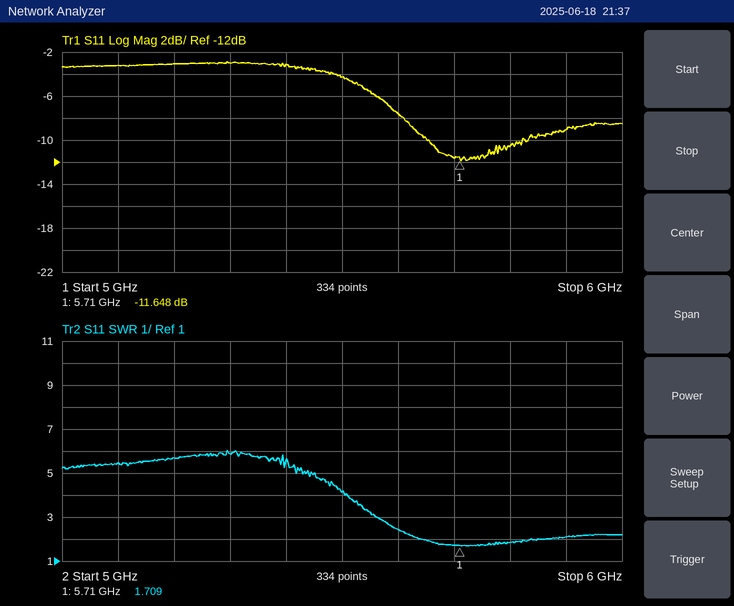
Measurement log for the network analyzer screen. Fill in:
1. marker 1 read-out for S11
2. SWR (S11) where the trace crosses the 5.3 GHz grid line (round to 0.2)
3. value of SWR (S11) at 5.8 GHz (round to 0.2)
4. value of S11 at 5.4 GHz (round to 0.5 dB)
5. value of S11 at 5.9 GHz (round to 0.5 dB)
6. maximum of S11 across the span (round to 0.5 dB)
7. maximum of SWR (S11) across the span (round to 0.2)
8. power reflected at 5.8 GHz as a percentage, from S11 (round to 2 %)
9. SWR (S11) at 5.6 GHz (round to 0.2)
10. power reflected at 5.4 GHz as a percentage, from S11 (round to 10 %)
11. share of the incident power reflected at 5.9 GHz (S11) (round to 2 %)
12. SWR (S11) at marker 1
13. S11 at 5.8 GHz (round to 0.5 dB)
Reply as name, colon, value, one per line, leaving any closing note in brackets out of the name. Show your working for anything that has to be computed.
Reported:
marker 1 read-out for S11: -11.648 dB
SWR (S11) where the trace crosses the 5.3 GHz grid line: 5.8
value of SWR (S11) at 5.8 GHz: 1.8
value of S11 at 5.4 GHz: -3.0 dB
value of S11 at 5.9 GHz: -9.0 dB
maximum of S11 across the span: -3.0 dB
maximum of SWR (S11) across the span: 6.0
power reflected at 5.8 GHz as a percentage, from S11: 10^(-10.5/10) ≈ 8.91 %, so 8 % to the nearest 2 %
SWR (S11) at 5.6 GHz: 2.4
power reflected at 5.4 GHz as a percentage, from S11: 10^(-3/10) ≈ 50 %
share of the incident power reflected at 5.9 GHz (S11): 10^(-9/10) ≈ 12.6 %, so 12 % to the nearest 2 %
SWR (S11) at marker 1: 1.709
S11 at 5.8 GHz: -10.5 dB
